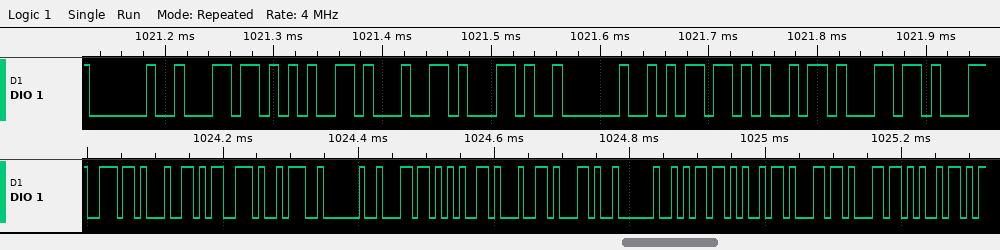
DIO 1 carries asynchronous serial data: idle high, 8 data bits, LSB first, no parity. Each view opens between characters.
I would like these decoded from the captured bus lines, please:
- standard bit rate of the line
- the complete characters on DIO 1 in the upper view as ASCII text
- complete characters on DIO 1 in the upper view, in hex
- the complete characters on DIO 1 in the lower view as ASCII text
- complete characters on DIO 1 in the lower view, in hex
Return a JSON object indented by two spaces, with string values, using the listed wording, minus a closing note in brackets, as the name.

{
  "standard bit rate of the line": "115200 baud",
  "the complete characters on DIO 1 in the upper view as ASCII text": "\" led, mil\"",
  "complete characters on DIO 1 in the upper view, in hex": "20, 6C, 65, 64, 2C, 20, 6D, 69, 6C",
  "the complete characters on DIO 1 in the lower view as ASCII text": "\"nds: led, milli\"",
  "complete characters on DIO 1 in the lower view, in hex": "6E, 64, 73, 3A, 20, 6C, 65, 64, 2C, 20, 6D, 69, 6C, 6C, 69"
}
